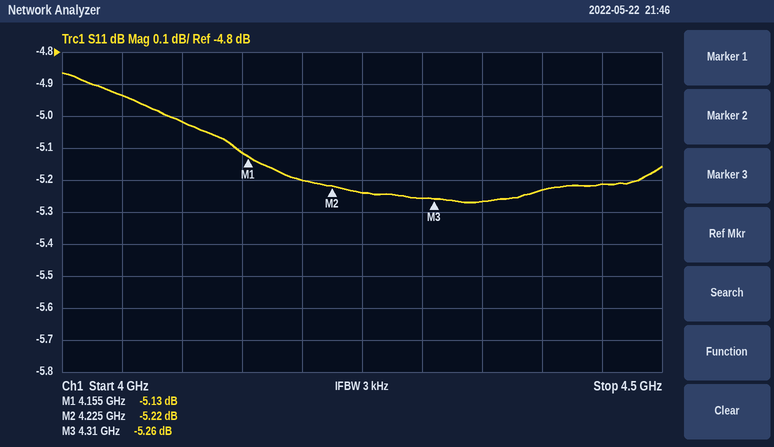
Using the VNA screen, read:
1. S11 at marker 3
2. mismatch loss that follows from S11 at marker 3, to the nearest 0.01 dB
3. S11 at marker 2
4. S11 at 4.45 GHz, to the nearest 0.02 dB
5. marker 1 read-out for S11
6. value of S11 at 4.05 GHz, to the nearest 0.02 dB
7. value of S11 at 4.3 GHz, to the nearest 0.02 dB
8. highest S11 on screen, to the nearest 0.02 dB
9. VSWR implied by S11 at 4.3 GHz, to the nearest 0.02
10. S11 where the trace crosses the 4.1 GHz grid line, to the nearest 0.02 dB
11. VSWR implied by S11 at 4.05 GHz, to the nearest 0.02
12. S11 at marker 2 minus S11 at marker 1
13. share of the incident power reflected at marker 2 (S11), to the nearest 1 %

-5.26 dB
1.54 dB
-5.22 dB
-5.22 dB
-5.13 dB
-4.94 dB
-5.26 dB
-4.86 dB
3.40
-5.02 dB
3.62
-0.09 dB
30 %
